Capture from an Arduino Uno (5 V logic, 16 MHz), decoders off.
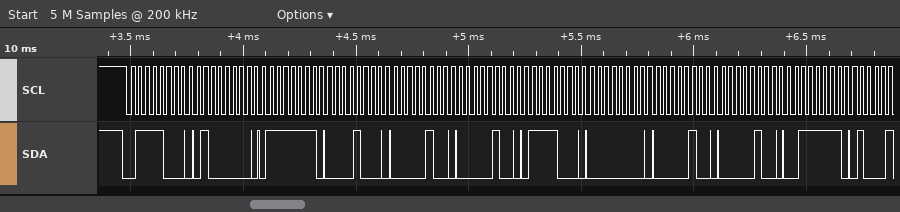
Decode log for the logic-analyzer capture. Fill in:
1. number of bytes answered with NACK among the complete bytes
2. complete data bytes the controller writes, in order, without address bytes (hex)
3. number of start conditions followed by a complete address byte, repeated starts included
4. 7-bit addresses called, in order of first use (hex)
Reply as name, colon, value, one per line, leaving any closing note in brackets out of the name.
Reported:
number of bytes answered with NACK among the complete bytes: 0
complete data bytes the controller writes, in order, without address bytes: 40 7F 08 04 04 78 00 04 04 3F
number of start conditions followed by a complete address byte, repeated starts included: 1
7-bit addresses called, in order of first use: 0x3C
